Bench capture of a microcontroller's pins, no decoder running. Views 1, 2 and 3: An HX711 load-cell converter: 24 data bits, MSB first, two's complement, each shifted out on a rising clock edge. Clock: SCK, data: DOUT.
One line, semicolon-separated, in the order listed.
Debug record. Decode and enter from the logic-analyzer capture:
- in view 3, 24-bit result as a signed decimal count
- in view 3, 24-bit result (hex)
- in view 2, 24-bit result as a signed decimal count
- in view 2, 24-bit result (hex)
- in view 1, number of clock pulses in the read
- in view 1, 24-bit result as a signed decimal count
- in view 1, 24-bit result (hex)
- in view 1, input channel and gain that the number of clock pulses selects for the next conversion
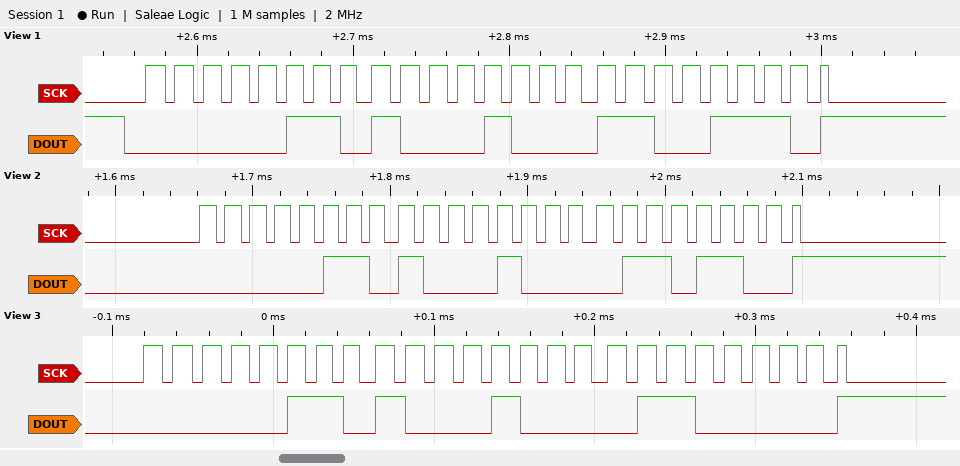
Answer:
428128; 0x068860; 428140; 0x06886C; 25; 428238; 0x0688CE; channel A, gain 128
